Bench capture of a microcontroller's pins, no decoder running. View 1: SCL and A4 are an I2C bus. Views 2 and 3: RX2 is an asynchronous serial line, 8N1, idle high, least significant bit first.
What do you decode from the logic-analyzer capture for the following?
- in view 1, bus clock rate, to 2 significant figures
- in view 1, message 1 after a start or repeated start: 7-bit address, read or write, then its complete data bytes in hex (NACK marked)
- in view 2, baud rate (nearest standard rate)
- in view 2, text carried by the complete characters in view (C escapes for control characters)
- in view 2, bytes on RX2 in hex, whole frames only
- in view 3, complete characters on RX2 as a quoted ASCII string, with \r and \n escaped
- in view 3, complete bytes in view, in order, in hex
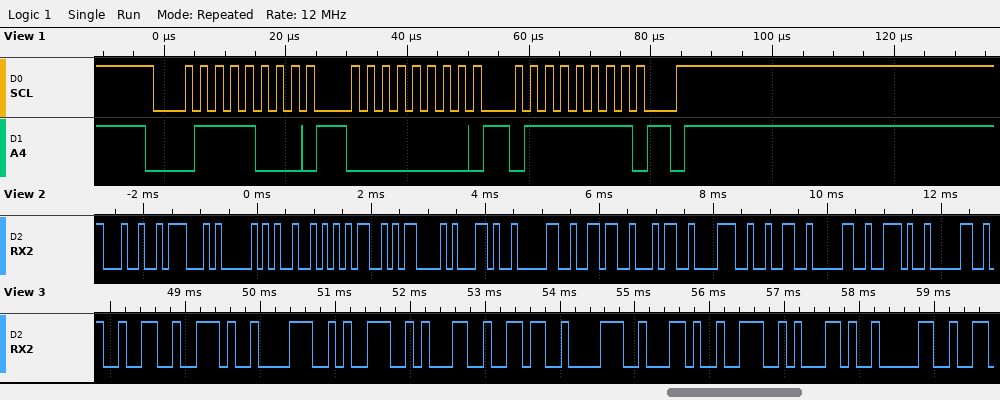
400 kHz
0x3C write: 00 7F
9600 baud
"$GPRMC,064820.0"
24 47 50 52 4D 43 2C 30 36 34 38 32 30 2E 30
"2.89168,N,0"
32 2E 38 39 31 36 38 2C 4E 2C 30
